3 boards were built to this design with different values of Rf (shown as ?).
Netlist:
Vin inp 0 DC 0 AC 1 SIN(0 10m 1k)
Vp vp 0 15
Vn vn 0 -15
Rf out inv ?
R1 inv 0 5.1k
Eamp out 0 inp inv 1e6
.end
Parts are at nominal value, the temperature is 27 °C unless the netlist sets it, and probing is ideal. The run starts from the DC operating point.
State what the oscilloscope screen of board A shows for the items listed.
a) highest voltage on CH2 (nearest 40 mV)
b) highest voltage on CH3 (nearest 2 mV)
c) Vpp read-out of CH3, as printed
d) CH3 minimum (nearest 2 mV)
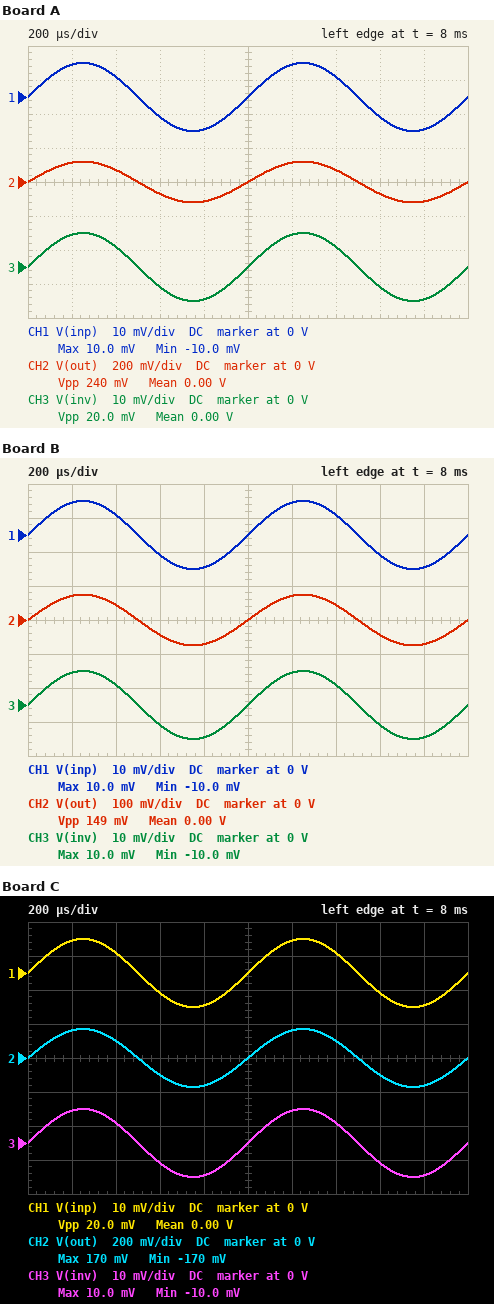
120 mV
10 mV
20.0 mV
-10 mV
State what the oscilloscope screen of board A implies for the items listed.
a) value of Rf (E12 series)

56 kΩ
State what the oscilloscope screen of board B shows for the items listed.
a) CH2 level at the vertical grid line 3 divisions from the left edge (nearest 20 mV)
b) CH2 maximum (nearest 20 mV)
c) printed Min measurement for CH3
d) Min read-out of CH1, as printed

-40 mV
80 mV
-10.0 mV
-10.0 mV
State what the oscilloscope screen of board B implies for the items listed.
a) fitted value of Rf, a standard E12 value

33 kΩ
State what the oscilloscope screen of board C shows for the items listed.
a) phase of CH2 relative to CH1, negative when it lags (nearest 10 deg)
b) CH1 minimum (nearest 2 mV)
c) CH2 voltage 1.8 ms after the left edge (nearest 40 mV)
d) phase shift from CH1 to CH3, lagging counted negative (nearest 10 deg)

0 deg
-10 mV
-160 mV
0 deg
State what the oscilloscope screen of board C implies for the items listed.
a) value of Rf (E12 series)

82 kΩ
